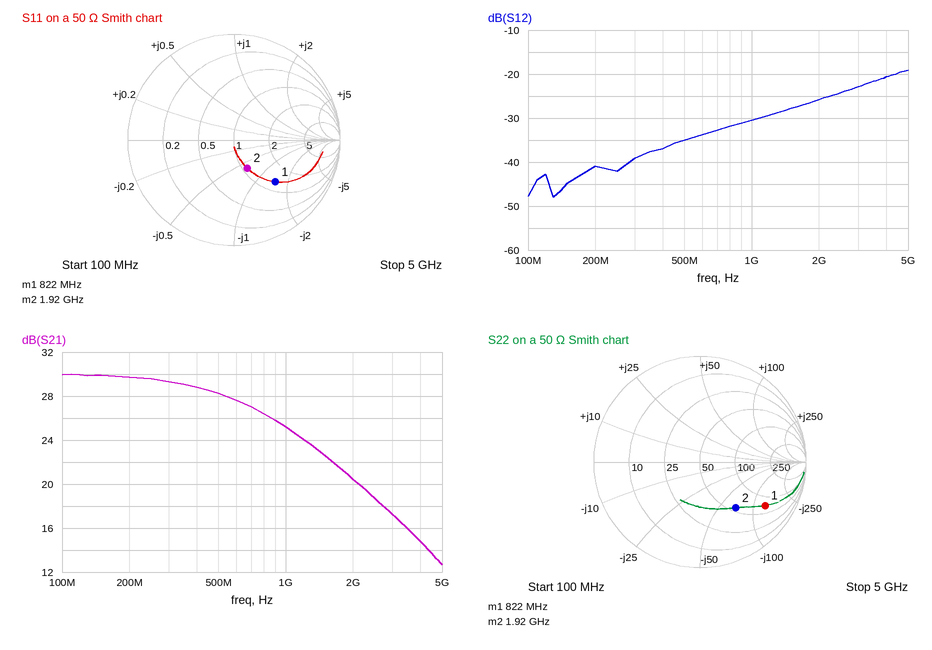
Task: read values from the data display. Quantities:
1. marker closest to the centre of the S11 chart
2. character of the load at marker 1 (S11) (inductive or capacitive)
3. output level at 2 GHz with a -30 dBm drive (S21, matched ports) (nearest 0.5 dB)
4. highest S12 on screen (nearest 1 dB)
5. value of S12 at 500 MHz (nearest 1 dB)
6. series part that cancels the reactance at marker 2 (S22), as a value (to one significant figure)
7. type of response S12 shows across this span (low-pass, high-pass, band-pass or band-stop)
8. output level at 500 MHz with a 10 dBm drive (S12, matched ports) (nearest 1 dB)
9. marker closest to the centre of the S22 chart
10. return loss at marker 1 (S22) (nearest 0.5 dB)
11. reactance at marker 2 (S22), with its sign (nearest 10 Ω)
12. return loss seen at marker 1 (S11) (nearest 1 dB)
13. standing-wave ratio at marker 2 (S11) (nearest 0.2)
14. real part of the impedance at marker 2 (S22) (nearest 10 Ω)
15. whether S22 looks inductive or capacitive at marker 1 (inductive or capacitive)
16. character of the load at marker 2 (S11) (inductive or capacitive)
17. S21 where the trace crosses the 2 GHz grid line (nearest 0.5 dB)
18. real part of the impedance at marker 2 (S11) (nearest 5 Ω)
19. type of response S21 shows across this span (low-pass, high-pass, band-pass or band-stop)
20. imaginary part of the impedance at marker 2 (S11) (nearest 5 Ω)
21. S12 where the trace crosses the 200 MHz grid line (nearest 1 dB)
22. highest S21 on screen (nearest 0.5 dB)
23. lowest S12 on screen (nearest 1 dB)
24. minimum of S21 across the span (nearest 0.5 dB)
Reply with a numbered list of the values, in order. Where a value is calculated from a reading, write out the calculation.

1. marker 2
2. capacitive
3. -30 dBm + (20.5 dB) = -9.5 dBm
4. -19 dB
5. -35 dB
6. L = 70 Ω/(2π × 1.92 GHz) ≈ 6 nH
7. high-pass
8. 10 dBm + (-35 dB) = -25 dBm
9. marker 2
10. 2.5 dB
11. -70 Ω
12. 5 dB
13. 1.8
14. 60 Ω
15. capacitive
16. capacitive
17. 20.5 dB
18. 55 Ω
19. low-pass
20. -30 Ω
21. -41 dB
22. 30.0 dB
23. -48 dB
24. 12.5 dB
